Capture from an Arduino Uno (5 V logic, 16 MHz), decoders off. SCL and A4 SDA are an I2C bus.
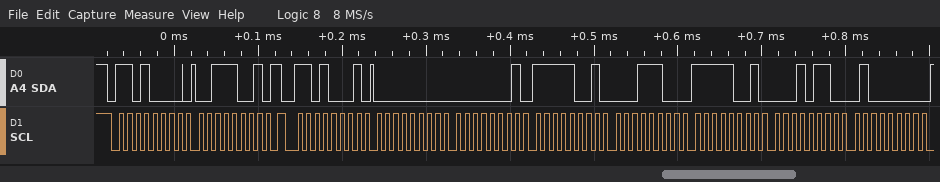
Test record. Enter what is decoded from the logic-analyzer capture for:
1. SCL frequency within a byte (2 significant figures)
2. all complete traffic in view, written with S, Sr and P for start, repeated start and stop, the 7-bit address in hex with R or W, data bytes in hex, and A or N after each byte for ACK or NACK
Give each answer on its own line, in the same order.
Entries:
100 kHz
S 68W A 39 A Sr 68R A 00 A 01 A F9 A 1C A F9 A 16 A 40 A
